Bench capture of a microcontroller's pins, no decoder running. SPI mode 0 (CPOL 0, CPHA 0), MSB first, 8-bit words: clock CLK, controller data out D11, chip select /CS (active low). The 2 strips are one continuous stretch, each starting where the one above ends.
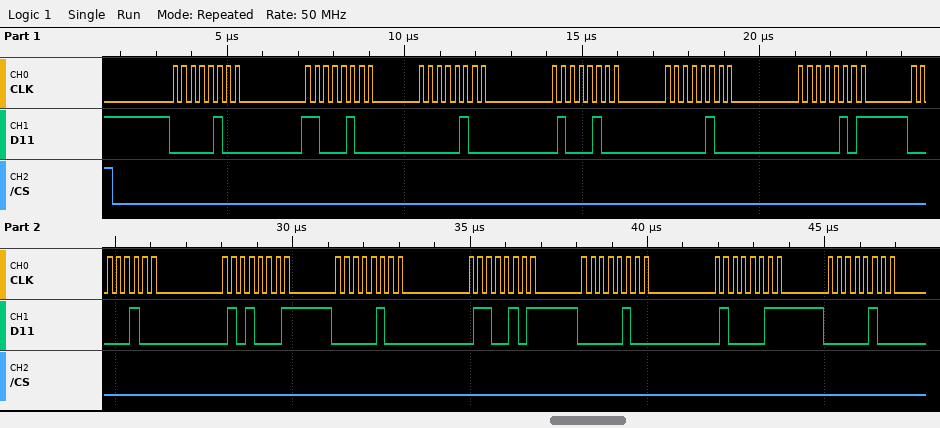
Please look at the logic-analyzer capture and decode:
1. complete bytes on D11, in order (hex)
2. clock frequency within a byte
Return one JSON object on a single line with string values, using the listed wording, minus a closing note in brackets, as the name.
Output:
{"complete bytes on D11, in order": "0x04 0xC4 0x04 0x44 0x04 0x05 0x04 0x51 0x04 0x65 0x04 0x43 0x04", "clock frequency within a byte": "4 MHz"}
